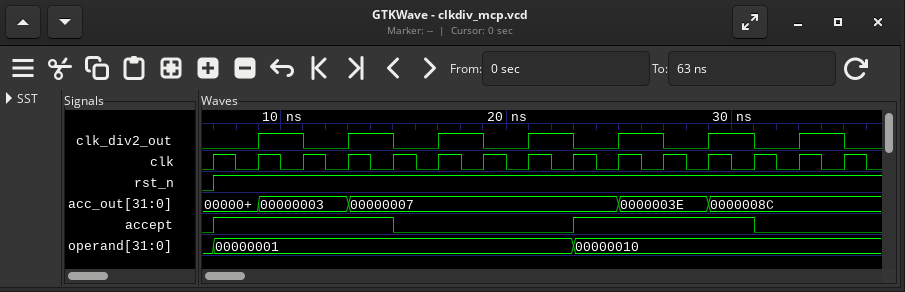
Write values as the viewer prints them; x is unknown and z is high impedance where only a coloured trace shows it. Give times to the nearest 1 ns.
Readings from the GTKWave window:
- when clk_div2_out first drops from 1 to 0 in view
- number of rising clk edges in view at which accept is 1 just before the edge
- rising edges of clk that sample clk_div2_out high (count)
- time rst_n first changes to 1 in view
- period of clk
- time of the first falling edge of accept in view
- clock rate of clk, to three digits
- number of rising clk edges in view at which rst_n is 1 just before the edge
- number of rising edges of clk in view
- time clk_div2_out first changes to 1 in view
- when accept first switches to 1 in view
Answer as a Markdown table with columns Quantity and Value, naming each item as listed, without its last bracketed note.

| Quantity | Value |
|---|---|
| when clk_div2_out first drops from 1 to 0 in view | 11 ns |
| number of rising clk edges in view at which accept is 1 just before the edge | 8 |
| rising edges of clk that sample clk_div2_out high | 7 |
| time rst_n first changes to 1 in view | 7 ns |
| period of clk | 2 ns |
| time of the first falling edge of accept in view | 15 ns |
| clock rate of clk, to three digits | 500 MHz |
| number of rising clk edges in view at which rst_n is 1 just before the edge | 14 |
| number of rising edges of clk in view | 15 |
| time clk_div2_out first changes to 1 in view | 9 ns |
| when accept first switches to 1 in view | 7 ns |
